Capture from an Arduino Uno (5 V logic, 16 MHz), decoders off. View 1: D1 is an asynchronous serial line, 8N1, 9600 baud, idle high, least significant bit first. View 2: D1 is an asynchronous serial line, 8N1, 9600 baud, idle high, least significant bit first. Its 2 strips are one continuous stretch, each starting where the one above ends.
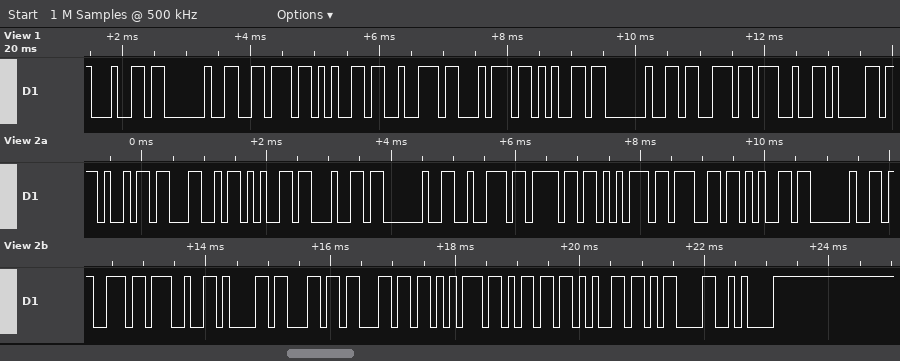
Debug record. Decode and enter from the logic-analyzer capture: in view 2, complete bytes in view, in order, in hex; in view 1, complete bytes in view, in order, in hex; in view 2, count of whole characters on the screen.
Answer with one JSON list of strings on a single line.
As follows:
["69 4C 65 64 20 72 6F 75 67 65 20 73 27 61 6C 6C 75 6D 65 0D 0A", "64 20 76 65 72 74 65 20 73 27 61", "21"]
